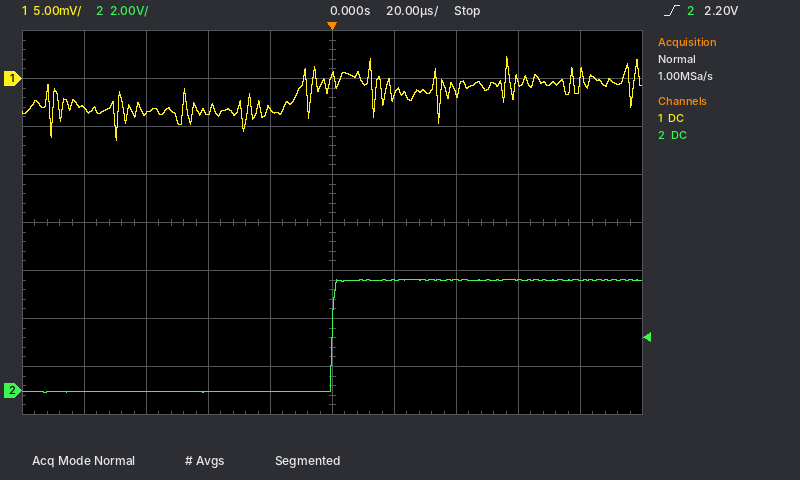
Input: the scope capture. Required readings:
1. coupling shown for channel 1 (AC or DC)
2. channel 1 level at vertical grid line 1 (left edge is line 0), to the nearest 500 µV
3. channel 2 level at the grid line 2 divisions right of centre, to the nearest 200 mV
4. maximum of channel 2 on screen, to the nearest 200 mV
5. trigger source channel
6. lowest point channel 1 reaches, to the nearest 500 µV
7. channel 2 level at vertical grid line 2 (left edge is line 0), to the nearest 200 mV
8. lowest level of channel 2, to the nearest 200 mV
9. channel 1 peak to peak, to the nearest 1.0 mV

DC
-3.0 mV
4.6 V
4.6 V
channel 2
-6.5 mV
0.0 V
0.0 V
9.0 mV
